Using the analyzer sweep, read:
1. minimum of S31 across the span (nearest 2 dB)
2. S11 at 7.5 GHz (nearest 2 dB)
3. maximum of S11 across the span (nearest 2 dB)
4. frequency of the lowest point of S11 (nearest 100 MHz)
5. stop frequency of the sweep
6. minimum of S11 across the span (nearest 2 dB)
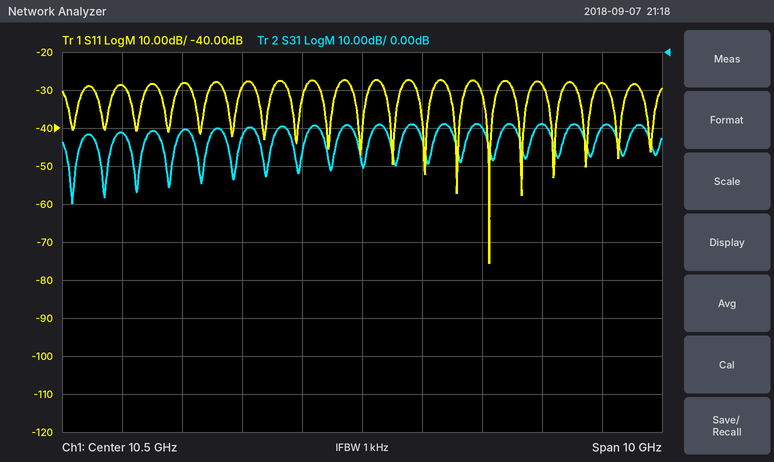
-40 dB
-28 dB
-28 dB
12.6 GHz
15.5 GHz
-76 dB
